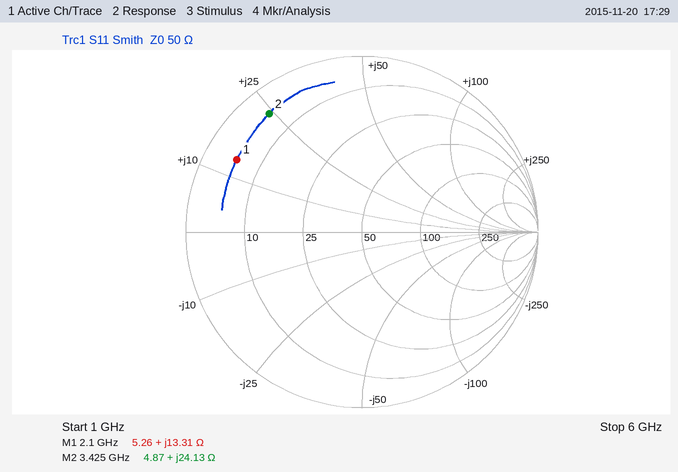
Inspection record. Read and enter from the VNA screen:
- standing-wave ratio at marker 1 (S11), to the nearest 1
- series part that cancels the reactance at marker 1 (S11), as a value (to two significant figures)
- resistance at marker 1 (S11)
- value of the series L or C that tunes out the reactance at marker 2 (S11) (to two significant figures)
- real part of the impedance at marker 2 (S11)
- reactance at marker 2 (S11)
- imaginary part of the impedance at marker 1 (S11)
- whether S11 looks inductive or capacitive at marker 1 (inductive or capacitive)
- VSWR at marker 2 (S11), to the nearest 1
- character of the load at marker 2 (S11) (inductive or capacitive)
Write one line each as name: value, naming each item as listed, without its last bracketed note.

standing-wave ratio at marker 1 (S11), to the nearest 1: 10
series part that cancels the reactance at marker 1 (S11), as a value: 5.7 pF
resistance at marker 1: 5.26 Ω
value of the series L or C that tunes out the reactance at marker 2 (S11): 1.9 pF
real part of the impedance at marker 2: 4.87 Ω
reactance at marker 2: +24.13 Ω
imaginary part of the impedance at marker 1: +13.31 Ω
whether S11 looks inductive or capacitive at marker 1: inductive
VSWR at marker 2 (S11), to the nearest 1: 13
character of the load at marker 2 (S11): inductive
